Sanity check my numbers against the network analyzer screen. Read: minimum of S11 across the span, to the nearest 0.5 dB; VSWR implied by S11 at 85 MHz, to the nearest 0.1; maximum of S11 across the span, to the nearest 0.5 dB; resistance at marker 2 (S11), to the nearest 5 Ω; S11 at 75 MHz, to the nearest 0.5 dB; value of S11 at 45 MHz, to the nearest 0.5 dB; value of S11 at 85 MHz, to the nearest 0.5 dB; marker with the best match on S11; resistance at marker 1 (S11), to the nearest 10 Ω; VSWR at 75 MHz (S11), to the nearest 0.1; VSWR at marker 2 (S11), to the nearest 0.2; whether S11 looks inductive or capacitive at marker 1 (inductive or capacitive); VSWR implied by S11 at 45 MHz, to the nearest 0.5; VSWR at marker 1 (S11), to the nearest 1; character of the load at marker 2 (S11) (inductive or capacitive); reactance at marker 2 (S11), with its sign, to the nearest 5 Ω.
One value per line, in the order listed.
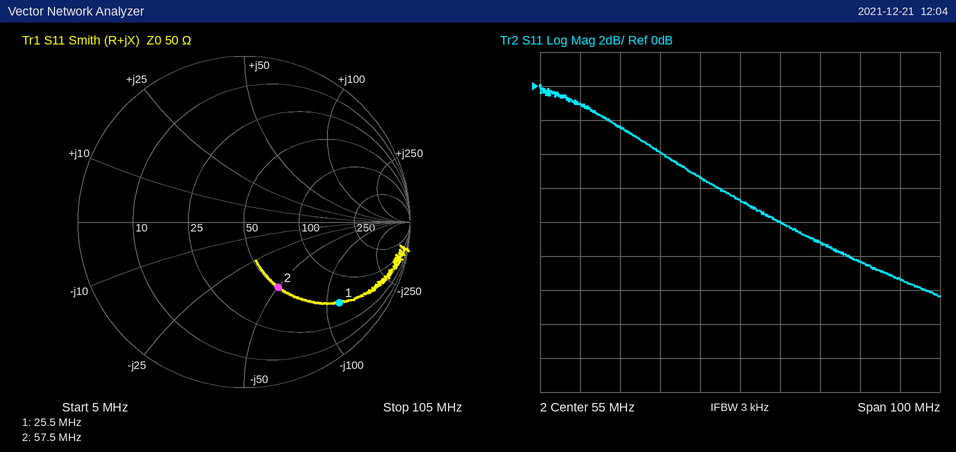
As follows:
-12.5 dB
1.9
0.0 dB
50 Ω
-9.0 dB
-5.5 dB
-10.5 dB
marker 2
50 Ω
2.1
2.6
capacitive
3.5
7
capacitive
-50 Ω
